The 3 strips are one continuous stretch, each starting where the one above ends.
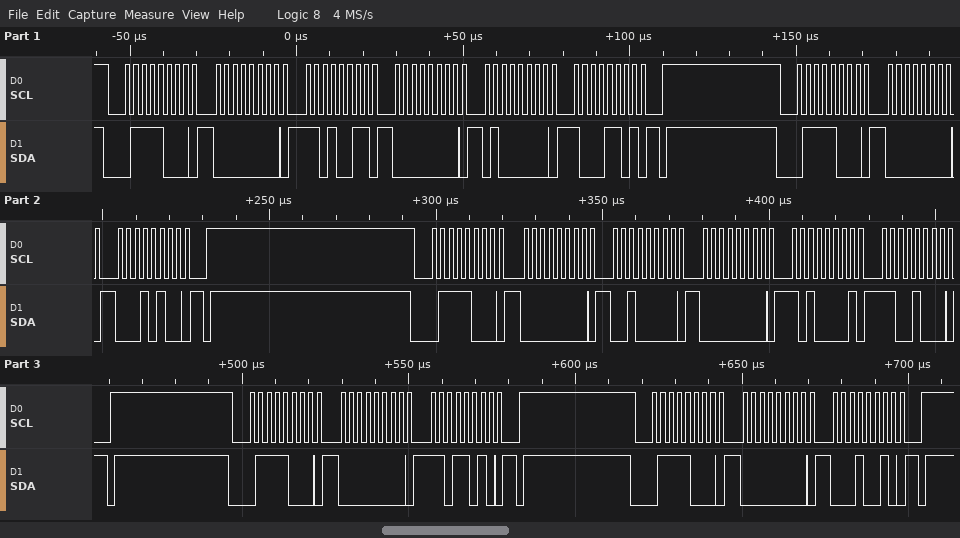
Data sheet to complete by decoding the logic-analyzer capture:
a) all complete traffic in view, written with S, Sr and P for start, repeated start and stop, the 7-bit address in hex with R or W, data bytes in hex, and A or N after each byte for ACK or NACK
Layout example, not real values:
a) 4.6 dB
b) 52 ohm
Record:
a) S 3CW A 00 A D3 A 00 A 40 A 8D A P S 3CW A 00 A 14 A P S 3CW A 00 A 20 A 00 A A1 A C8 A P S 3CW A 00 A DA A P S 3CW A 00 A 12 A P
